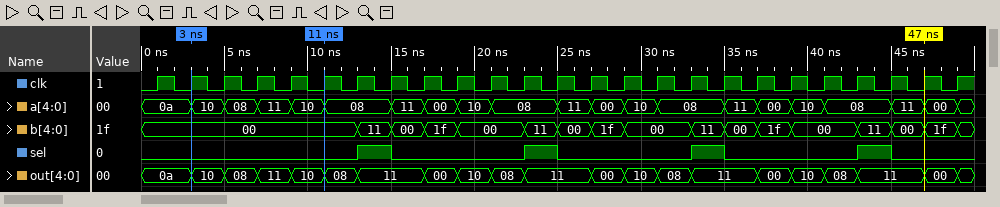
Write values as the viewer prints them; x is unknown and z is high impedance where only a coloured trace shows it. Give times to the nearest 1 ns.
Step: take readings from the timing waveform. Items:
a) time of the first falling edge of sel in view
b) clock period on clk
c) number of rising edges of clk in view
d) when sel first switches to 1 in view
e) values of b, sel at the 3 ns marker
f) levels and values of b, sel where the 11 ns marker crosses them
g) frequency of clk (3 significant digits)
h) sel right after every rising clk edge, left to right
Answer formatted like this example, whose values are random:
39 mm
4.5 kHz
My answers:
15 ns
2 ns
25
13 ns
b=00, sel=0
b=00, sel=0
500 MHz
0 0 0 0 0 0 1 0 0 0 0 1 0 0 0 0 1 0 0 0 0 1 0 0 0
